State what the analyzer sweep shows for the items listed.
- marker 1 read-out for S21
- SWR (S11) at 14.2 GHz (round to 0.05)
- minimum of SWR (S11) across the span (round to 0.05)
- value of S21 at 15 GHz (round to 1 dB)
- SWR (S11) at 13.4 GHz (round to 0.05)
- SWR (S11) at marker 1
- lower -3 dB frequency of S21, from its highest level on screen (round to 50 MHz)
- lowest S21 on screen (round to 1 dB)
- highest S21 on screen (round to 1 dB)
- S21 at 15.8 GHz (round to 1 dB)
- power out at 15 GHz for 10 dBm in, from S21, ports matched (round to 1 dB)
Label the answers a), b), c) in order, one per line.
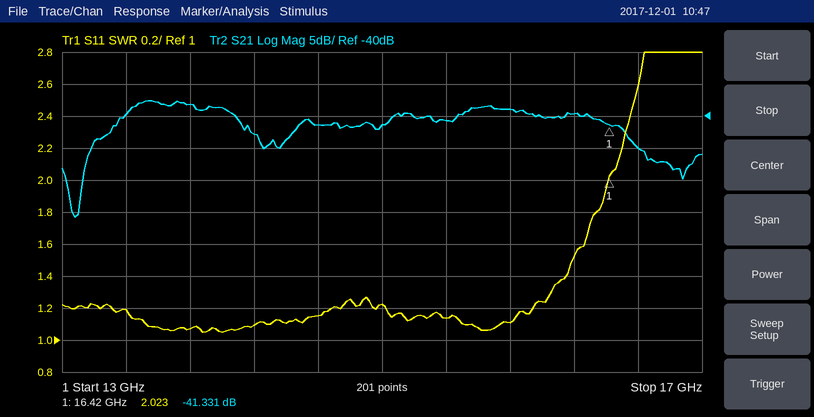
a) -41.331 dB
b) 1.10
c) 1.05
d) -41 dB
e) 1.20
f) 2.023
g) 13.35 GHz
h) -56 dB
i) -38 dB
j) -39 dB
k) -31 dBm
